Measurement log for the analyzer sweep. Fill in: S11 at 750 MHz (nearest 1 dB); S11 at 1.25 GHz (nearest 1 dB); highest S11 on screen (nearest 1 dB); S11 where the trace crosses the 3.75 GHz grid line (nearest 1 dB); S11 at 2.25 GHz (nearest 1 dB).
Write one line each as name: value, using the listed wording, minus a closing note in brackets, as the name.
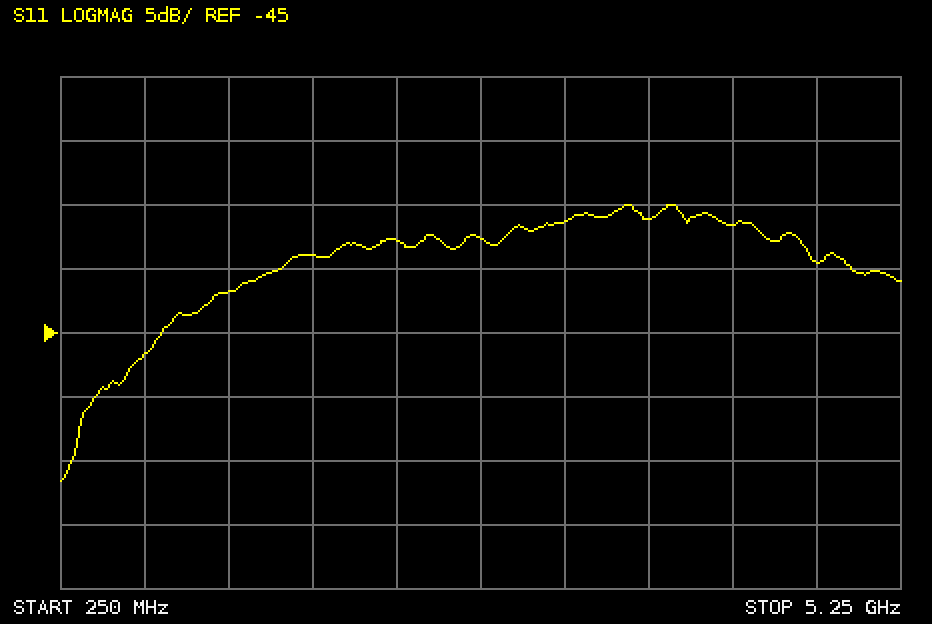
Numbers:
S11 at 750 MHz: -47 dB
S11 at 1.25 GHz: -42 dB
highest S11 on screen: -35 dB
S11 where the trace crosses the 3.75 GHz grid line: -36 dB
S11 at 2.25 GHz: -38 dB
